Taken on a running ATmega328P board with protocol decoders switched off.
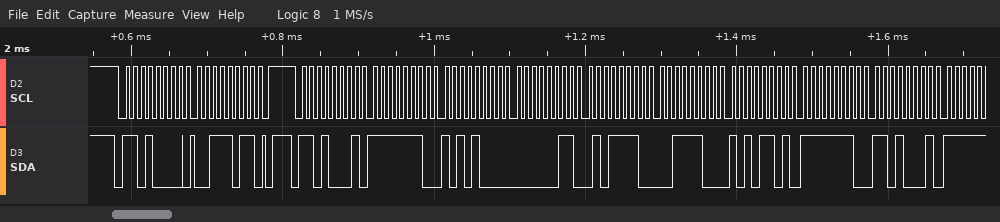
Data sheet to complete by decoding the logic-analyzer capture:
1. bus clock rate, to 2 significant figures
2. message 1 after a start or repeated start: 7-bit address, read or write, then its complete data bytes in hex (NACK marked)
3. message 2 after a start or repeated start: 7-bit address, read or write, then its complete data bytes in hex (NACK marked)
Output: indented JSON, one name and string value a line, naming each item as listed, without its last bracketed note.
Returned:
{
  "bus clock rate, to 2 significant figures": "100 kHz",
  "message 1 after a start or repeated start: 7-bit address, read or write, then its complete data bytes in hex": "0x68 write: 3B",
  "message 2 after a start or repeated start: 7-bit address, read or write, then its complete data bytes in hex": "0x68 read: FE A8 03 5E 3C AD FE D1"
}
